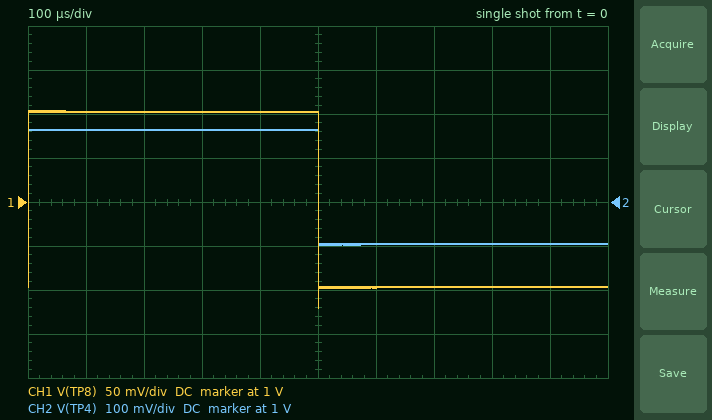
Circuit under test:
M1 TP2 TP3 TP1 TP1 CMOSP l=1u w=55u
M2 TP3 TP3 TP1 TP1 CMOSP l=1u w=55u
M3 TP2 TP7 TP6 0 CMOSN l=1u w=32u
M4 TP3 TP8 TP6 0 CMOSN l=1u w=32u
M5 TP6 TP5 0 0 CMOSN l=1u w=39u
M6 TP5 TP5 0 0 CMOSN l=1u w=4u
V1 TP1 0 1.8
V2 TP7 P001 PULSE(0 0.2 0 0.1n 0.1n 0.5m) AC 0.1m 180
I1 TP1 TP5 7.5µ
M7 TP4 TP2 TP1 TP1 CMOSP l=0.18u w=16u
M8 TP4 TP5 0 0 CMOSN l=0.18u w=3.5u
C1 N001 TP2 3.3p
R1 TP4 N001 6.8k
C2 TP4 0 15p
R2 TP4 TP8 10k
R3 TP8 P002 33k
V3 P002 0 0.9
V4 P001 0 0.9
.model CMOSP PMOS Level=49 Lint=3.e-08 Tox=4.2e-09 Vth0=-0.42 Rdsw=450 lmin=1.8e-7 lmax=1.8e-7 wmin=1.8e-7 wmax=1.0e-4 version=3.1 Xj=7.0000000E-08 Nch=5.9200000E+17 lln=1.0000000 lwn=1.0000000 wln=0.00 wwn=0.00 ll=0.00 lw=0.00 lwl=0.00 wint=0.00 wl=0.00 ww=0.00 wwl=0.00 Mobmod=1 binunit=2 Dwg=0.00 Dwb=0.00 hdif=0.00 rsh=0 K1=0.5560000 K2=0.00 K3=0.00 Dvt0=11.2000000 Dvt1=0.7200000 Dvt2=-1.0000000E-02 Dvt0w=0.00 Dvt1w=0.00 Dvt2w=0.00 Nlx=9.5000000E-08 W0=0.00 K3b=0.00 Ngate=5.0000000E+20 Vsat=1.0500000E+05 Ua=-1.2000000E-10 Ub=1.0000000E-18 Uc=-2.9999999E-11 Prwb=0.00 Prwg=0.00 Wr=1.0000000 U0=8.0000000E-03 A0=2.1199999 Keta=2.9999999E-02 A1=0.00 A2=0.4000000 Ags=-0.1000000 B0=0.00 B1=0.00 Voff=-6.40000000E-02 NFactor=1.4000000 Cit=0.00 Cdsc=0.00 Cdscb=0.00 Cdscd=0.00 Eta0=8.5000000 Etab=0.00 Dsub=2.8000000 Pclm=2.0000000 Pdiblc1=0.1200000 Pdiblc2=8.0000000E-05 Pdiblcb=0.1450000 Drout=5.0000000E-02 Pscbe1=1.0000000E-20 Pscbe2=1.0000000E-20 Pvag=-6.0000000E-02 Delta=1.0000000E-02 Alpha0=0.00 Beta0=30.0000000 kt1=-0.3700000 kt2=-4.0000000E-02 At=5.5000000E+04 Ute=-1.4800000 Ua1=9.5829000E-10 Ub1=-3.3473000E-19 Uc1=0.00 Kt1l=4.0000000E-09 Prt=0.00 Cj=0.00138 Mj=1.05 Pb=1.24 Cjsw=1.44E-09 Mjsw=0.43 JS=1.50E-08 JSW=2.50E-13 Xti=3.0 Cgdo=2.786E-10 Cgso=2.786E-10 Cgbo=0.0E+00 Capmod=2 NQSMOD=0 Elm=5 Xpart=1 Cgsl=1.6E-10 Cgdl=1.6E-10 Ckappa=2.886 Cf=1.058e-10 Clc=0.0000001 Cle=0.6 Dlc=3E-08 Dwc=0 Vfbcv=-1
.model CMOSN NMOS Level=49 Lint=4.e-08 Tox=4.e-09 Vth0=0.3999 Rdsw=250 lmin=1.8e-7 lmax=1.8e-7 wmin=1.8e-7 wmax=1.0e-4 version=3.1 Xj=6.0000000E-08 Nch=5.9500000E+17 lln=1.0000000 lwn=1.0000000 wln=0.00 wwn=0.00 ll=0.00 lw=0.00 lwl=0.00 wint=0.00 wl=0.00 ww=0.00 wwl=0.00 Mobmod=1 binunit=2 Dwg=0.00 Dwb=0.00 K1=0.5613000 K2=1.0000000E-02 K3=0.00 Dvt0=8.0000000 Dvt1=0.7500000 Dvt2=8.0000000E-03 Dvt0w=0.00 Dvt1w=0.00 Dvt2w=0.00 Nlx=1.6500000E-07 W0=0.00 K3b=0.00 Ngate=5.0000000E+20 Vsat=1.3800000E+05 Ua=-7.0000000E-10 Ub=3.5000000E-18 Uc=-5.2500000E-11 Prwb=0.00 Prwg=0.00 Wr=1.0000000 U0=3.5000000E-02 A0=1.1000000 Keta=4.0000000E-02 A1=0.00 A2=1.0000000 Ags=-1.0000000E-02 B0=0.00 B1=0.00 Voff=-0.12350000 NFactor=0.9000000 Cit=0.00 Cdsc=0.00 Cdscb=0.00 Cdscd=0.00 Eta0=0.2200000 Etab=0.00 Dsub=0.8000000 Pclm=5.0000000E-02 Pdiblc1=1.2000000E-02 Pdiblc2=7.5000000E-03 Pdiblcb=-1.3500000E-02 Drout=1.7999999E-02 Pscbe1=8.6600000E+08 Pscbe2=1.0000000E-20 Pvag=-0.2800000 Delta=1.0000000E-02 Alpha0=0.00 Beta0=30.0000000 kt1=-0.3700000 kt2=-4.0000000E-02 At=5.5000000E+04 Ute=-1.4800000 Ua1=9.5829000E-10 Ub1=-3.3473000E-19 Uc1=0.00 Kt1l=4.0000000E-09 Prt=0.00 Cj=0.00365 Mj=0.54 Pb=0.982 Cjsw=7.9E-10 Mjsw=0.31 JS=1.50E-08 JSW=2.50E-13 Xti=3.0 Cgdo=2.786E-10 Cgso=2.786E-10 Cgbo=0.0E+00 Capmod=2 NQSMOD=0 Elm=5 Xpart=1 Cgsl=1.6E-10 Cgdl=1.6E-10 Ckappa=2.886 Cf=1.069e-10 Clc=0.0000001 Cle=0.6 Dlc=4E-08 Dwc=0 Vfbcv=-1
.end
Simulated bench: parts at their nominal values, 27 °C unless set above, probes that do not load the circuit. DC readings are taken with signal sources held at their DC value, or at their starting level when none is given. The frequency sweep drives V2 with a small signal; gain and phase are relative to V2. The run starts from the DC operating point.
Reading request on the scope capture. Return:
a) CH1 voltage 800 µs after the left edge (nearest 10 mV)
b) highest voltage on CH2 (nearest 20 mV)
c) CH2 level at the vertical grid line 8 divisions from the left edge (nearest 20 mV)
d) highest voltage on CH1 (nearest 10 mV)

900 mV
1.16 V
900 mV
1.10 V
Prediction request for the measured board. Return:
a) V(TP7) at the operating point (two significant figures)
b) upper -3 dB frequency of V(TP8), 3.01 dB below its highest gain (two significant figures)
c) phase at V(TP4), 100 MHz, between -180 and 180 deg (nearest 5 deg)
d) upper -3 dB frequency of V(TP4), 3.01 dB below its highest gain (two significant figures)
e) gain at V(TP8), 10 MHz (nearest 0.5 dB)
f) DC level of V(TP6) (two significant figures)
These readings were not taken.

900 mV
46 MHz
-160 deg
58 MHz
-1.5 dB
310 mV
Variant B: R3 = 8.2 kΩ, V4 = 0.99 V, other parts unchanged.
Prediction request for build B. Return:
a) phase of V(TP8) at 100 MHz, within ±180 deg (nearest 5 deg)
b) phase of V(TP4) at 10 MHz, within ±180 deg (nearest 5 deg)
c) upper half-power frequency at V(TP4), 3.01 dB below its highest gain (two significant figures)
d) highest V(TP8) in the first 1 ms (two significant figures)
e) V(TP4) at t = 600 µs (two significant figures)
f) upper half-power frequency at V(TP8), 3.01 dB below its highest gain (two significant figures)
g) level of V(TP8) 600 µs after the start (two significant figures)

105 deg
-30 deg
14 MHz
1.2 V
1.1 V
12 MHz
990 mV
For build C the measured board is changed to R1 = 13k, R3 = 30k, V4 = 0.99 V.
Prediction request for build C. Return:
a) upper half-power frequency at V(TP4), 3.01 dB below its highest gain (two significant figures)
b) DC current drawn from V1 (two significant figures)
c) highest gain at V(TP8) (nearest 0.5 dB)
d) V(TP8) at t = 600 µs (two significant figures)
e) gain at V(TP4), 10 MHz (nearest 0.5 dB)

63 MHz
210 µA
6.0 dB
990 mV
1.5 dB
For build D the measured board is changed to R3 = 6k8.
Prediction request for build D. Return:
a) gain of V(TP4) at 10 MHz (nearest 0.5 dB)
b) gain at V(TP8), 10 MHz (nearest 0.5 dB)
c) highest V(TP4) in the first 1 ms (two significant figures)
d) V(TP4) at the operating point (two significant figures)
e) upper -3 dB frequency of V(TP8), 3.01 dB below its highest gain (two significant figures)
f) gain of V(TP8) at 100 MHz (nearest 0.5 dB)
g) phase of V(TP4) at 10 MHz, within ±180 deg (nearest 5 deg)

5.0 dB
-3.0 dB
1.4 V
910 mV
9.8 MHz
-17.0 dB
-30 deg
